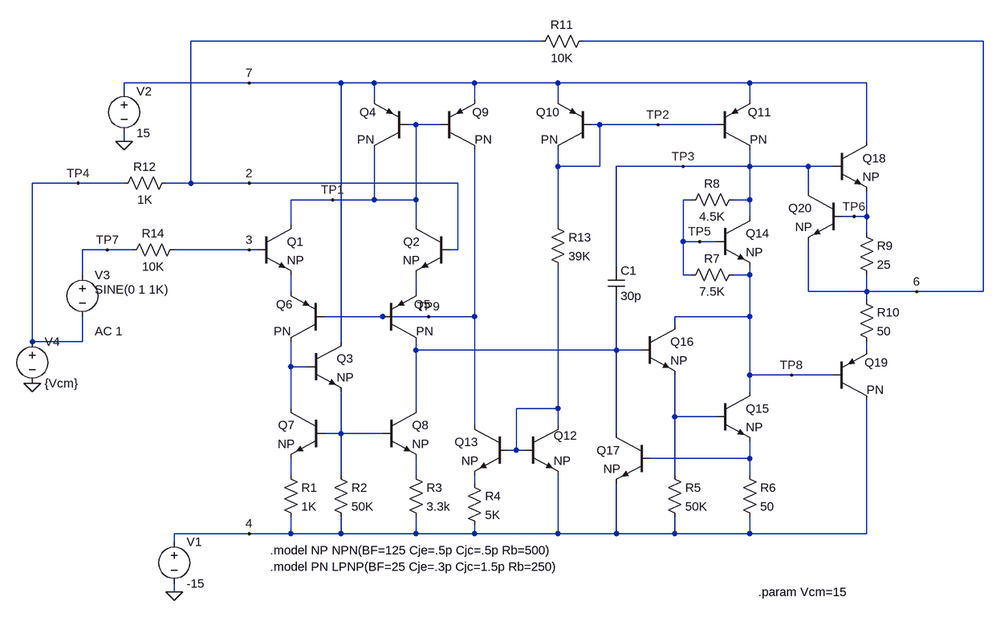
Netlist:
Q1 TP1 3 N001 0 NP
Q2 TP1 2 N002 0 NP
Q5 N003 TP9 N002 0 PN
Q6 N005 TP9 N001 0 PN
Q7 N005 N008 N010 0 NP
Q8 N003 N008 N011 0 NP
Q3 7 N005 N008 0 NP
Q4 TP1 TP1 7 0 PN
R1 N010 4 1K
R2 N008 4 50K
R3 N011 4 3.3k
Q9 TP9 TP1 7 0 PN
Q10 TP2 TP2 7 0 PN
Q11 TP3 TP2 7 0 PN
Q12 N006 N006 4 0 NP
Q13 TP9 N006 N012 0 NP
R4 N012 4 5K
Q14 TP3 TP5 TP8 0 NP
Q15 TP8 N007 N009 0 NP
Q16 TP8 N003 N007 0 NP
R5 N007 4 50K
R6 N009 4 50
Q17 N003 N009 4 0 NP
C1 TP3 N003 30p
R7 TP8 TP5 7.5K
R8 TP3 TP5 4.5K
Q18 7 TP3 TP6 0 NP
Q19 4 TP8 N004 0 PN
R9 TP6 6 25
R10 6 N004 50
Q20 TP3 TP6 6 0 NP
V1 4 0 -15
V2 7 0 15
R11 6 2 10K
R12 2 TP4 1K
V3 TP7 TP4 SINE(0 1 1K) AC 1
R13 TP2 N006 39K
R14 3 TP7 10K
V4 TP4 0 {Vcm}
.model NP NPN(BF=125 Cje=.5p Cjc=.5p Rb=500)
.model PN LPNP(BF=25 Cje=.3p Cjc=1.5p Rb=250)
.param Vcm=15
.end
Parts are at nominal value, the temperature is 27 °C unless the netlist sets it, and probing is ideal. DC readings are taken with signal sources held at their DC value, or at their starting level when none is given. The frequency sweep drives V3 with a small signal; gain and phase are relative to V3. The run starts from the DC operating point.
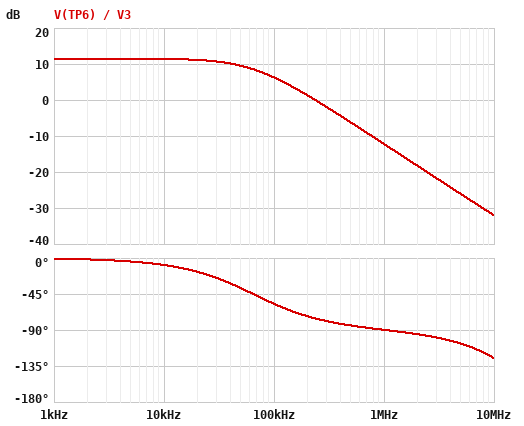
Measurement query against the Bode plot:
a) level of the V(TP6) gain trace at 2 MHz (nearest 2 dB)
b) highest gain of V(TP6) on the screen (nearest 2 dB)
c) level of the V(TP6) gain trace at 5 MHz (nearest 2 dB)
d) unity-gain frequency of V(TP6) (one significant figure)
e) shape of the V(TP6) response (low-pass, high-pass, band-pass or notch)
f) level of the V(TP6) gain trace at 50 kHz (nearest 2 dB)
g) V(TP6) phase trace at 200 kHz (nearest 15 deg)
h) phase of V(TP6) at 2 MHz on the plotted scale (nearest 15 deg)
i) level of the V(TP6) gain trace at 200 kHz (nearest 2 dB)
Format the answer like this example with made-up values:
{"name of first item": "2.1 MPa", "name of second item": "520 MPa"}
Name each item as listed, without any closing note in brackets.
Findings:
{"level of the V(TP6) gain trace at 2 MHz": "-18 dB", "highest gain of V(TP6) on the screen": "12 dB", "level of the V(TP6) gain trace at 5 MHz": "-26 dB", "unity-gain frequency of V(TP6)": "200 kHz", "shape of the V(TP6) response": "low-pass", "level of the V(TP6) gain trace at 50 kHz": "10 dB", "V(TP6) phase trace at 200 kHz": "-75 deg", "phase of V(TP6) at 2 MHz on the plotted scale": "-90 deg", "level of the V(TP6) gain trace at 200 kHz": "2 dB"}
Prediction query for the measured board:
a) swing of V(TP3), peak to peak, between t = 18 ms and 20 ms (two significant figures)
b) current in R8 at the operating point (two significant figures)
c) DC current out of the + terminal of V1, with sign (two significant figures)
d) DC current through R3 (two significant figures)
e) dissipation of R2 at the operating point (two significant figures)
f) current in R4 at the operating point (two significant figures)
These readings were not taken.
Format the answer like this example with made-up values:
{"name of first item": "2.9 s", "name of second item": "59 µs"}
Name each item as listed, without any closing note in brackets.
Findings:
{"swing of V(TP3), peak to peak, between t = 18 ms and 20 ms": "11 V", "current in R8 at the operating point": "110 µA", "DC current out of the + terminal of V1, with sign": "-1.5 mA", "DC current through R3": "8.8 µA", "dissipation of R2 at the operating point": "9.3 µW", "current in R4 at the operating point": "19 µA"}
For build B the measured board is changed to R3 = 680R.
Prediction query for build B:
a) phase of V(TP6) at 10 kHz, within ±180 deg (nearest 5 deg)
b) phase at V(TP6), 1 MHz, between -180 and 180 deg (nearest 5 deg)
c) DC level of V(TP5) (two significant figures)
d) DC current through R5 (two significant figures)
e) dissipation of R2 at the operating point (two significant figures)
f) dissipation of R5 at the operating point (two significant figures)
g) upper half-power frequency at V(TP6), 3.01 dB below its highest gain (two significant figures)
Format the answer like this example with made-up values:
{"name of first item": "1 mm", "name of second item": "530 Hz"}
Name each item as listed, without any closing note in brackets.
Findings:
{"phase of V(TP6) at 10 kHz, within ±180 deg": "0 deg", "phase at V(TP6), 1 MHz, between -180 and 180 deg": "-45 deg", "DC level of V(TP5)": "15 V", "DC current through R5": "14 µA", "dissipation of R2 at the operating point": "9.1 µW", "dissipation of R5 at the operating point": "10 µW", "upper half-power frequency at V(TP6), 3.01 dB below its highest gain": "1.4 MHz"}
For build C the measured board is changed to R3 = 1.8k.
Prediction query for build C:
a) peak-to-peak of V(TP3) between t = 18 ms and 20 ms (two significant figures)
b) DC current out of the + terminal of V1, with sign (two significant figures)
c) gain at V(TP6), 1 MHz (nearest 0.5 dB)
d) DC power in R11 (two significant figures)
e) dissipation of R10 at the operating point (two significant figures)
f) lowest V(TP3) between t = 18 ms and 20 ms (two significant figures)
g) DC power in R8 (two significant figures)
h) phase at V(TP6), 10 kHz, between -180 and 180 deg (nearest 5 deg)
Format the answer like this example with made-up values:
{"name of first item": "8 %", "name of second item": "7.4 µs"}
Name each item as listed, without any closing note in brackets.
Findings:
{"peak-to-peak of V(TP3) between t = 18 ms and 20 ms": "11 V", "DC current out of the + terminal of V1, with sign": "-1.2 mA", "gain at V(TP6), 1 MHz": "-8.5 dB", "DC power in R11": "25 µW", "dissipation of R10 at the operating point": "130 nW", "lowest V(TP3) between t = 18 ms and 20 ms": "4.3 V", "DC power in R8": "46 µW", "phase at V(TP6), 10 kHz, between -180 and 180 deg": "-5 deg"}
